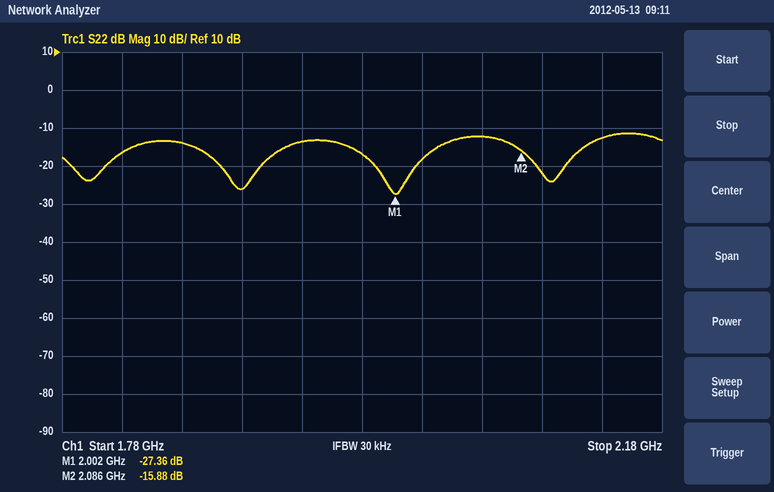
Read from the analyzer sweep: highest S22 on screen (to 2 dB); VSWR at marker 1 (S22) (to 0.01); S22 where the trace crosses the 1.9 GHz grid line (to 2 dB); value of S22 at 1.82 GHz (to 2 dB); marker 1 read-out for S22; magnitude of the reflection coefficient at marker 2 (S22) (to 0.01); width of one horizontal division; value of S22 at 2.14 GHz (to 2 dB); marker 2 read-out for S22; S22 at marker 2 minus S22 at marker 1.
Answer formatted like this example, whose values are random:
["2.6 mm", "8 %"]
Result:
["-12 dB", "1.09", "-26 dB", "-16 dB", "-27.36 dB", "0.16", "40 MHz", "-12 dB", "-15.88 dB", "11.48 dB"]
